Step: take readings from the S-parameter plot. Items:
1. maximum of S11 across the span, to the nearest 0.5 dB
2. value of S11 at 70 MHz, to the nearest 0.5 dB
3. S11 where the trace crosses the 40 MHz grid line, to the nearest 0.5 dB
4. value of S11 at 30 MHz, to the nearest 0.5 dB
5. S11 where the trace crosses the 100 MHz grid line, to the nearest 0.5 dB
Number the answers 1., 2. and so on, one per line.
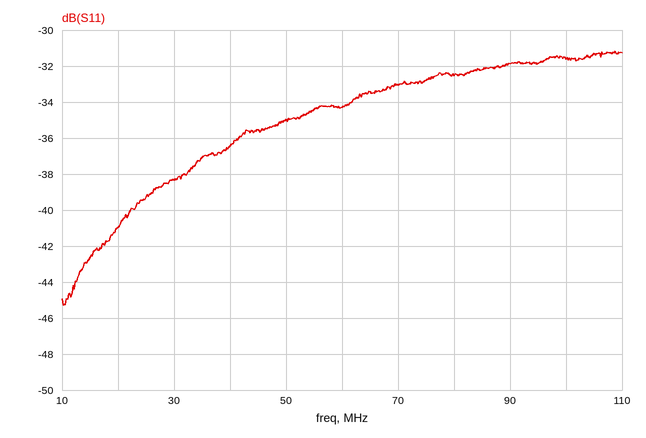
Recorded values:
1. -31.0 dB
2. -33.0 dB
3. -36.5 dB
4. -38.5 dB
5. -31.5 dB
